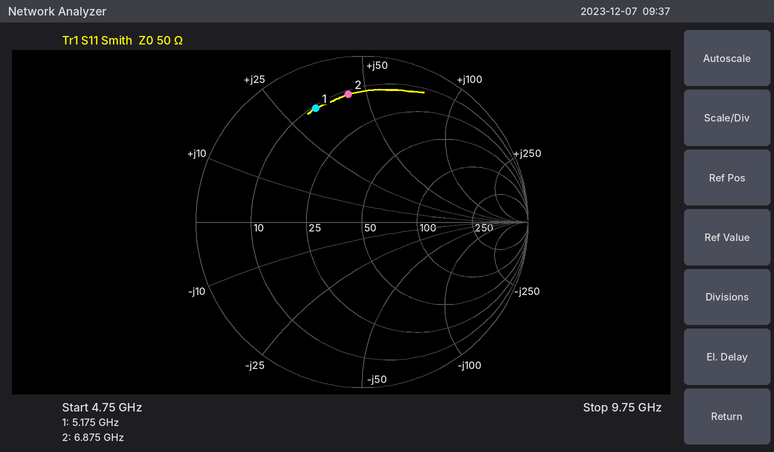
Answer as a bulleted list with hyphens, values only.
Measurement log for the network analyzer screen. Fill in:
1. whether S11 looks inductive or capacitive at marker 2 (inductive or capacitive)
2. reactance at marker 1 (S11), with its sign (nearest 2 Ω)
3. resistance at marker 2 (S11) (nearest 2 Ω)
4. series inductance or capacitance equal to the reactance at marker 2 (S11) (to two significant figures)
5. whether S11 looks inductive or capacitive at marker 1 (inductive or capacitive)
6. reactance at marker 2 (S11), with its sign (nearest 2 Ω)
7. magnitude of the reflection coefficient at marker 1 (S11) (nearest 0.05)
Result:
- inductive
- +32 Ω
- 12 Ω
- 1.0 nH
- inductive
- +44 Ω
- 0.75
